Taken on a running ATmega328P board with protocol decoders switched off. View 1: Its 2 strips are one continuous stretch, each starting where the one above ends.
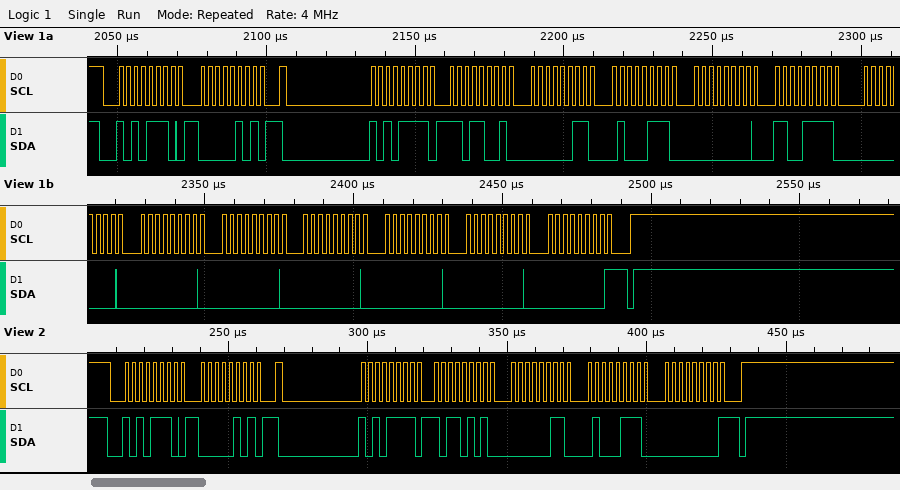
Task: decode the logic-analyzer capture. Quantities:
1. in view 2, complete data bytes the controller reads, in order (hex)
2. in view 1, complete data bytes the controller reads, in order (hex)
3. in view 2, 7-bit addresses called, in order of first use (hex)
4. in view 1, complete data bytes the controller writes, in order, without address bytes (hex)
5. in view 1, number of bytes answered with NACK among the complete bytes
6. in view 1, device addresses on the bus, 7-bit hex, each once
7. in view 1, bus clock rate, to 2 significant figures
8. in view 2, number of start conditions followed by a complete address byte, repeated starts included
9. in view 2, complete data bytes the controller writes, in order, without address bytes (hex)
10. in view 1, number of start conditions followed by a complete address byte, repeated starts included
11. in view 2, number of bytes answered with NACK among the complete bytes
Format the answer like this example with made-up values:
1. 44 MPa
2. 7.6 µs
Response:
1. B5 03 47 00
2. D9 03 47 00 CF 00 00 00 00 00 00 00
3. 0x57
4. 05
5. 1
6. 0x57
7. 400 kHz
8. 2
9. 05
10. 2
11. 1
